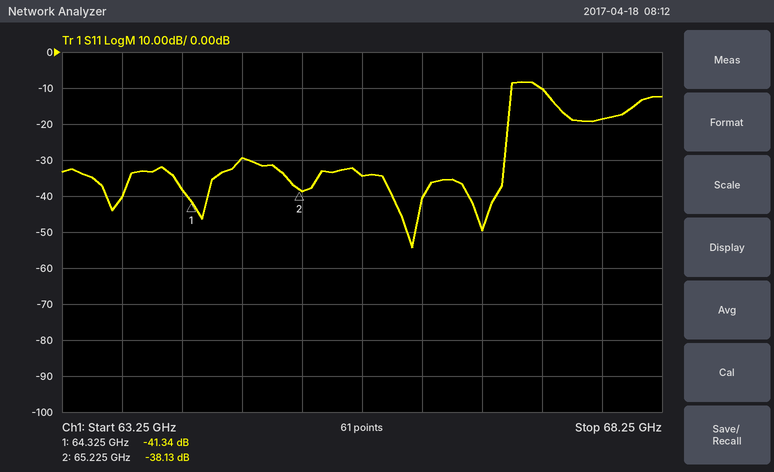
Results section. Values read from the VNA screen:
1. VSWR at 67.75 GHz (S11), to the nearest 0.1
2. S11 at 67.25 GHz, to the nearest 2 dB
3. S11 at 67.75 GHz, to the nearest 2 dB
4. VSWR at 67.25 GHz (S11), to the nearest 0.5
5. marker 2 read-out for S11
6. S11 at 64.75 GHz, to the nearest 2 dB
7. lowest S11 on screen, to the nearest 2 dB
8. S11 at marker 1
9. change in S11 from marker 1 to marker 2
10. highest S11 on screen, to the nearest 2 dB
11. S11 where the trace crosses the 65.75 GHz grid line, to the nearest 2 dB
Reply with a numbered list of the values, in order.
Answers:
1. 1.3
2. -10 dB
3. -18 dB
4. 2.0
5. -38.13 dB
6. -30 dB
7. -54 dB
8. -41.34 dB
9. 3.21 dB
10. -8 dB
11. -34 dB
